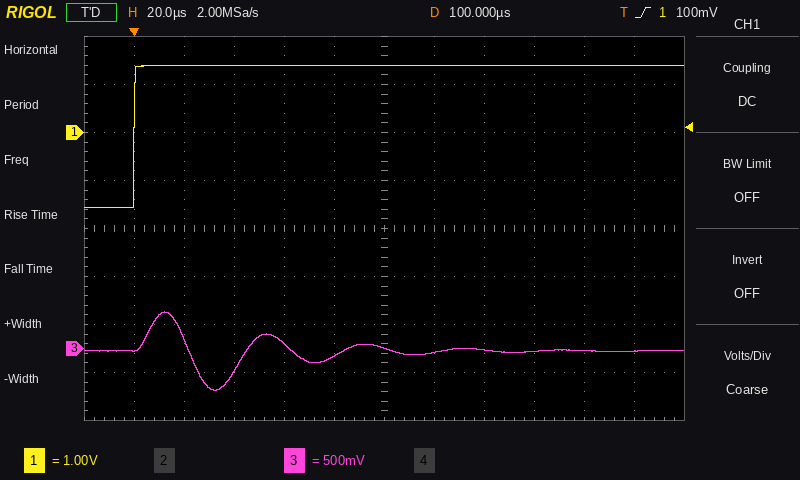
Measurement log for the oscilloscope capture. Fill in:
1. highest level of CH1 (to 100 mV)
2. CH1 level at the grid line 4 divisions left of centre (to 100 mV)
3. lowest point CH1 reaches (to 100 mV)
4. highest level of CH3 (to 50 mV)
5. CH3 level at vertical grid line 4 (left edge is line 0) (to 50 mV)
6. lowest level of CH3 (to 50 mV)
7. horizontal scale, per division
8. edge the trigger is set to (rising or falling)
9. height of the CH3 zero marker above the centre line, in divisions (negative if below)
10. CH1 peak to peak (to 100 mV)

1.4 V
1.4 V
-1.6 V
400 mV
50 mV
-450 mV
20 µs
rising
-2.5 div
3.0 V
